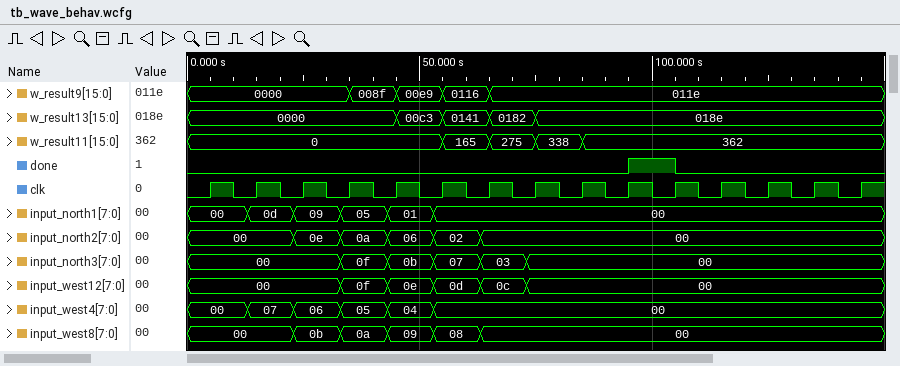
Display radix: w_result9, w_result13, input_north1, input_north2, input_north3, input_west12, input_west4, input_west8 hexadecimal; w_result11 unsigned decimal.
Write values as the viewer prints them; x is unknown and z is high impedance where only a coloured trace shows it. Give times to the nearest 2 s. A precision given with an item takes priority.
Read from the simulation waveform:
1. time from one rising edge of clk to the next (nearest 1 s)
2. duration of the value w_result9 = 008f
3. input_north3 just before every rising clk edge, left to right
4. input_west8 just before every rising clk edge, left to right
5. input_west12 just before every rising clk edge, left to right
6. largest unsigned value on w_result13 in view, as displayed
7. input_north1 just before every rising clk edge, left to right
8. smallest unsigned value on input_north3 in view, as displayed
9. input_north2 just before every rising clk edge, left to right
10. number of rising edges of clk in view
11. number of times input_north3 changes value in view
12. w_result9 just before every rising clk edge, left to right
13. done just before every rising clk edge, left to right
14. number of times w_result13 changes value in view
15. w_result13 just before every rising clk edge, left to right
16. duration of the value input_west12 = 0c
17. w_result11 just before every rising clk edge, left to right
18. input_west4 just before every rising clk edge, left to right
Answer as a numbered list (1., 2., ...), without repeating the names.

1. 10 s
2. 10 s
3. 00, 00, 00, 0f, 0b, 07, 03, 00, 00, 00, 00, 00, 00, 00, 00
4. 00, 00, 0b, 0a, 09, 08, 00, 00, 00, 00, 00, 00, 00, 00, 00
5. 00, 00, 00, 0f, 0e, 0d, 0c, 00, 00, 00, 00, 00, 00, 00, 00
6. 018e
7. 00, 0d, 09, 05, 01, 00, 00, 00, 00, 00, 00, 00, 00, 00, 00
8. 00
9. 00, 00, 0e, 0a, 06, 02, 00, 00, 00, 00, 00, 00, 00, 00, 00
10. 15
11. 5
12. 0000, 0000, 0000, 0000, 008f, 00e9, 0116, 011e, 011e, 011e, 011e, 011e, 011e, 011e, 011e
13. 0 0 0 0 0 0 0 0 0 0 1 0 0 0 0
14. 4
15. 0000, 0000, 0000, 0000, 0000, 00c3, 0141, 0182, 018e, 018e, 018e, 018e, 018e, 018e, 018e
16. 10 s
17. 0, 0, 0, 0, 0, 0, 165, 275, 338, 362, 362, 362, 362, 362, 362
18. 00, 07, 06, 05, 04, 00, 00, 00, 00, 00, 00, 00, 00, 00, 00
